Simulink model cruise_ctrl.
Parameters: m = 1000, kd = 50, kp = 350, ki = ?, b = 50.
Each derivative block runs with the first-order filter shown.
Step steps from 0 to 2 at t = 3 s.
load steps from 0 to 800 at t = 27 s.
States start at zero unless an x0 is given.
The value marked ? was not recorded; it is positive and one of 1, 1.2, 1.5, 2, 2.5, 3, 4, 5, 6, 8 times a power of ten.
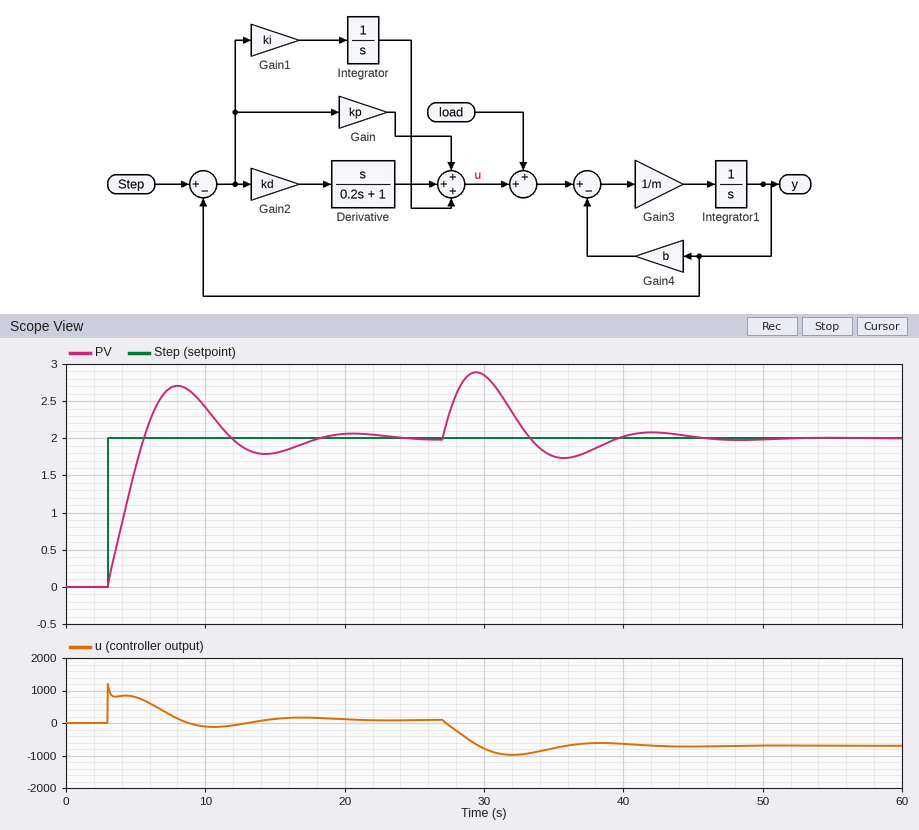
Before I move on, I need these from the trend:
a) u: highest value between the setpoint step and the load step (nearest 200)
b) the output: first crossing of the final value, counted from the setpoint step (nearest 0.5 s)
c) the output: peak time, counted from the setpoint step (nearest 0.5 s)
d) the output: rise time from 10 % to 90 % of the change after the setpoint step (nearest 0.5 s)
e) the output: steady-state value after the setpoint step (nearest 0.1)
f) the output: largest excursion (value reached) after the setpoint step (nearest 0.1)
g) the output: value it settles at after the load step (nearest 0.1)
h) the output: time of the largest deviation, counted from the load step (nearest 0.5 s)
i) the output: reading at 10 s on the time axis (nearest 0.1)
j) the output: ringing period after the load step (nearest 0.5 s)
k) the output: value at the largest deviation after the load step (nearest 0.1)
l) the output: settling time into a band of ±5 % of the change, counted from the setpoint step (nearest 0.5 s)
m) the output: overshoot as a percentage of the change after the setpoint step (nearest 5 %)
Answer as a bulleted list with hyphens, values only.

- 1200
- 2.5 s
- 5.0 s
- 2.0 s
- 2.0
- 2.7
- 2.0
- 2.5 s
- 2.4
- 12.5 s
- 2.9
- 13.5 s
- 35 %
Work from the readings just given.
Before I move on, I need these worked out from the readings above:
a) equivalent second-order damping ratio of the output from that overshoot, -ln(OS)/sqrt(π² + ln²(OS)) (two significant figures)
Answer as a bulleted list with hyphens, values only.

- 0.32
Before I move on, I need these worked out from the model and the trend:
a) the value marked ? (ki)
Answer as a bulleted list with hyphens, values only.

- 300
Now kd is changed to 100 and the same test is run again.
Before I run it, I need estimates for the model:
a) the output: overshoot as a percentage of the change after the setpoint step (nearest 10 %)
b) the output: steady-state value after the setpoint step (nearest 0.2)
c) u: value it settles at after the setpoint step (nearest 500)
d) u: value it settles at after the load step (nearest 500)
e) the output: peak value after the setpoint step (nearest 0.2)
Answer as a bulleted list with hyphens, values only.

- 30 %
- 2.0
- 0
- -500
- 2.6
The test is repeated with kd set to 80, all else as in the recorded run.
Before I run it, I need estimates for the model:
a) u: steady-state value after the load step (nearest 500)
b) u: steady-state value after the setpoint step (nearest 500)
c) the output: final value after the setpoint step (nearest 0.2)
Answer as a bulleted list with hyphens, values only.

- -500
- 0
- 2.0
